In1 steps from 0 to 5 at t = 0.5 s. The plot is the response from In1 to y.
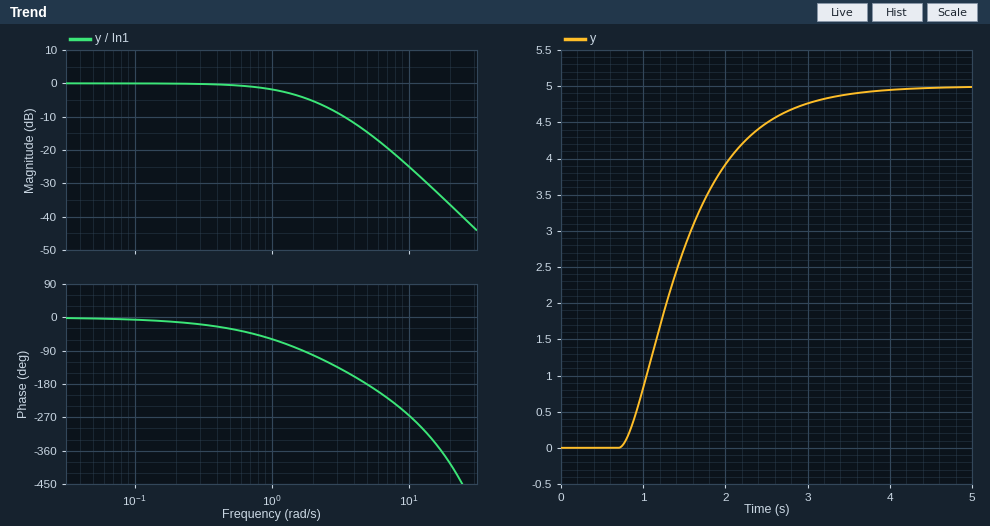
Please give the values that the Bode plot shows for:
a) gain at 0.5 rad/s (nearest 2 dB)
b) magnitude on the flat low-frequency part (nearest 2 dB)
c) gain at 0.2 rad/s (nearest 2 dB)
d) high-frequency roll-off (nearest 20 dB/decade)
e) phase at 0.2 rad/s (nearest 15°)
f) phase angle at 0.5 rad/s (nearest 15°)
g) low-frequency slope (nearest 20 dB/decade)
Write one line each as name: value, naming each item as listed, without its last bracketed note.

gain at 0.5 rad/s: 0 dB
magnitude on the flat low-frequency part: 0 dB
gain at 0.2 rad/s: 0 dB
high-frequency roll-off: -40 dB/decade
phase at 0.2 rad/s: -15°
phase angle at 0.5 rad/s: -30°
low-frequency slope: 0 dB/decade
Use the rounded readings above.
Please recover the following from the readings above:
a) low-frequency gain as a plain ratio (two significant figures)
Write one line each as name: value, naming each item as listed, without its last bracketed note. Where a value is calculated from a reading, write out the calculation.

low-frequency gain as a plain ratio: 10^(0 / 20) = 1.0
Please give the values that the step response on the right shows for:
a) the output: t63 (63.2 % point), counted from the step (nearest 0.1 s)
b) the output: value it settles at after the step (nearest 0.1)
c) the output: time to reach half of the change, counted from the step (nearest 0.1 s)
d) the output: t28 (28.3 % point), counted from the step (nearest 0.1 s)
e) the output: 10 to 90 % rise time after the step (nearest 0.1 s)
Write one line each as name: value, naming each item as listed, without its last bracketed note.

the output: t63 (63.2 % point), counted from the step: 1.1 s
the output: value it settles at after the step: 5.0
the output: time to reach half of the change, counted from the step: 0.9 s
the output: t28 (28.3 % point), counted from the step: 0.6 s
the output: 10 to 90 % rise time after the step: 1.6 s
